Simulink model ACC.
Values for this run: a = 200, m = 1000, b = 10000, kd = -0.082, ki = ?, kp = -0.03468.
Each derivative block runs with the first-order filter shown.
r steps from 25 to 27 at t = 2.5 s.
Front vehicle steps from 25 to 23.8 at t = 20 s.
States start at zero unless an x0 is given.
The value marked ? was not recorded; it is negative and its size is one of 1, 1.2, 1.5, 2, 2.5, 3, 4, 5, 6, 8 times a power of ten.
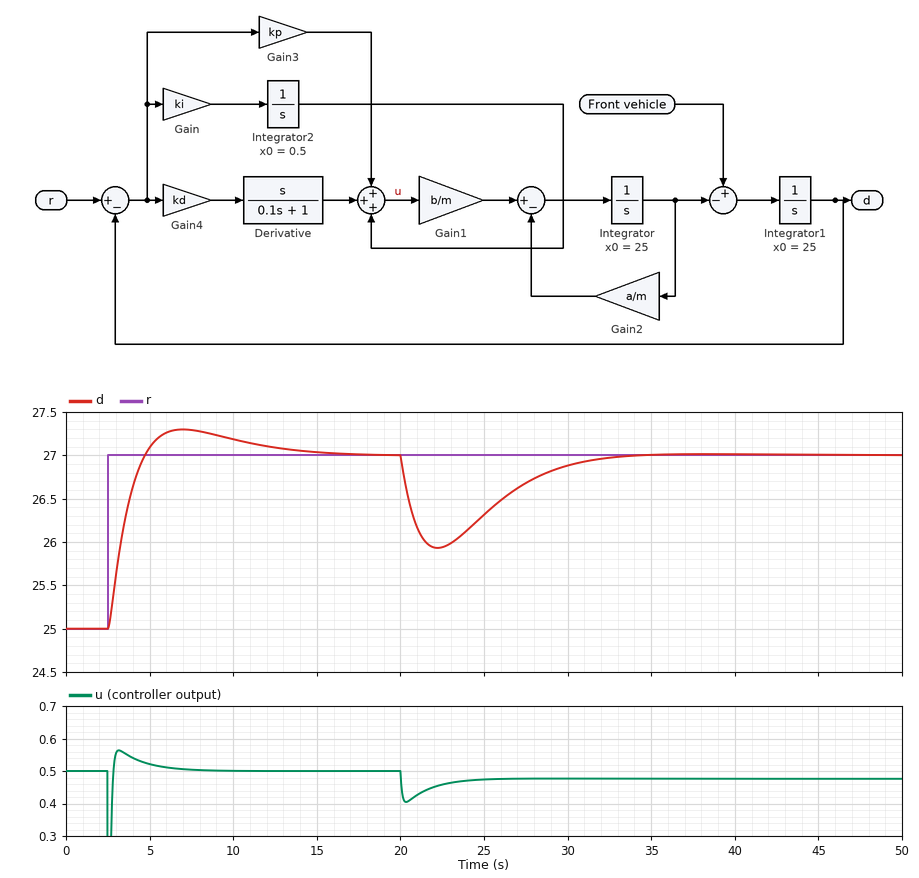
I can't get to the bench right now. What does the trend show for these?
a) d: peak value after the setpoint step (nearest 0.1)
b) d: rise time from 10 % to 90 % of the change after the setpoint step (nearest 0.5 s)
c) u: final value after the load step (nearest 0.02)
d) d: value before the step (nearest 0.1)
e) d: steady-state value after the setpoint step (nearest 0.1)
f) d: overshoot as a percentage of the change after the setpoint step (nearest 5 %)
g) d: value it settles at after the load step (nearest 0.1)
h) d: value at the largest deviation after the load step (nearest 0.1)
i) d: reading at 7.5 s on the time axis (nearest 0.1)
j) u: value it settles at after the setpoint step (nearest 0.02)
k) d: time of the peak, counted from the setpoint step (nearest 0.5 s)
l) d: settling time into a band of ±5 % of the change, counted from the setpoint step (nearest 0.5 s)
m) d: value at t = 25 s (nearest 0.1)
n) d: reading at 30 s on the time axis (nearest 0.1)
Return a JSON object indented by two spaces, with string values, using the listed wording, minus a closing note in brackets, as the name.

{
  "d: peak value after the setpoint step": "27.3",
  "d: rise time from 10 % to 90 % of the change after the setpoint step": "1.5 s",
  "u: final value after the load step": "0.48",
  "d: value before the step": "25.0",
  "d: steady-state value after the setpoint step": "27.0",
  "d: overshoot as a percentage of the change after the setpoint step": "15 %",
  "d: value it settles at after the load step": "27.0",
  "d: value at the largest deviation after the load step": "25.9",
  "d: reading at 7.5 s on the time axis": "27.3",
  "u: value it settles at after the setpoint step": "0.50",
  "d: time of the peak, counted from the setpoint step": "4.5 s",
  "d: settling time into a band of ±5 % of the change, counted from the setpoint step": "9.5 s",
  "d: value at t = 25 s": "26.3",
  "d: reading at 30 s on the time axis": "26.9"
}
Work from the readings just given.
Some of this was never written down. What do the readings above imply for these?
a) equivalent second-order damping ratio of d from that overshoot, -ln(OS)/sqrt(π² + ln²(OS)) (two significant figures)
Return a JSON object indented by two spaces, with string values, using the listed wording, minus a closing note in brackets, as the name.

{
  "equivalent second-order damping ratio of d from that overshoot, -ln(OS)/sqrt(π² + ln²(OS))": "0.52"
}
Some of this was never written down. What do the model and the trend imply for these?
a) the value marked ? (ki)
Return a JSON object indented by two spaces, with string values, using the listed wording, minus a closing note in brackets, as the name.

{
  "the value marked ?": "-0.004"
}
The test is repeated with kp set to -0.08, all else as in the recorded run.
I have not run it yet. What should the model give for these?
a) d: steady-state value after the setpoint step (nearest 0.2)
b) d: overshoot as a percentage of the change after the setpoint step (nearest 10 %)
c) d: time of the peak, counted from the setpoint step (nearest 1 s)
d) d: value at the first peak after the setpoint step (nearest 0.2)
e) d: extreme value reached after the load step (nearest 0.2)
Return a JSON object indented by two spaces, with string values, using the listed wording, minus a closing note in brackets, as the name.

{
  "d: steady-state value after the setpoint step": "27.0",
  "d: overshoot as a percentage of the change after the setpoint step": "20 %",
  "d: time of the peak, counted from the setpoint step": "3 s",
  "d: value at the first peak after the setpoint step": "27.4",
  "d: extreme value reached after the load step": "26.2"
}
